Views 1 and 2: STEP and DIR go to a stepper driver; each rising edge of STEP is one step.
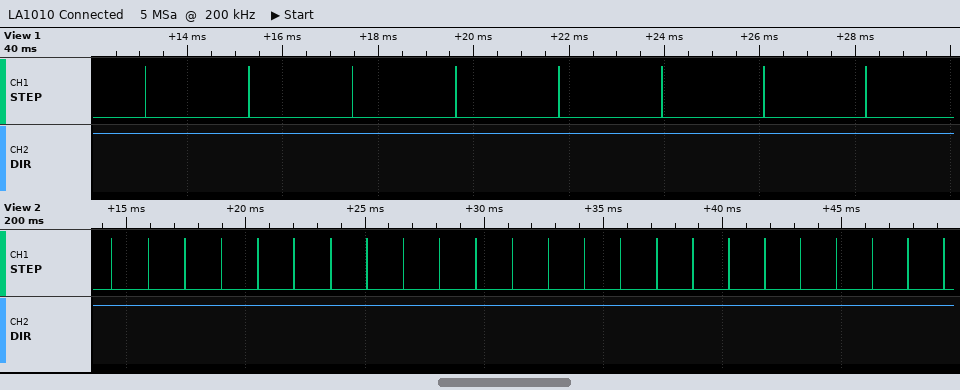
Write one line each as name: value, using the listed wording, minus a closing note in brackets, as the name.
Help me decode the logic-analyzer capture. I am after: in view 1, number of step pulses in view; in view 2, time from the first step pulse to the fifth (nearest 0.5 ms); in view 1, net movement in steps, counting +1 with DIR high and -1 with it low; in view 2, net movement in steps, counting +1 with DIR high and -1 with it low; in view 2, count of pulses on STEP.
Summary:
in view 1, number of step pulses in view: 8
in view 2, time from the first step pulse to the fifth: 6.0 ms
in view 1, net movement in steps, counting +1 with DIR high and -1 with it low: +8
in view 2, net movement in steps, counting +1 with DIR high and -1 with it low: +24
in view 2, count of pulses on STEP: 24
